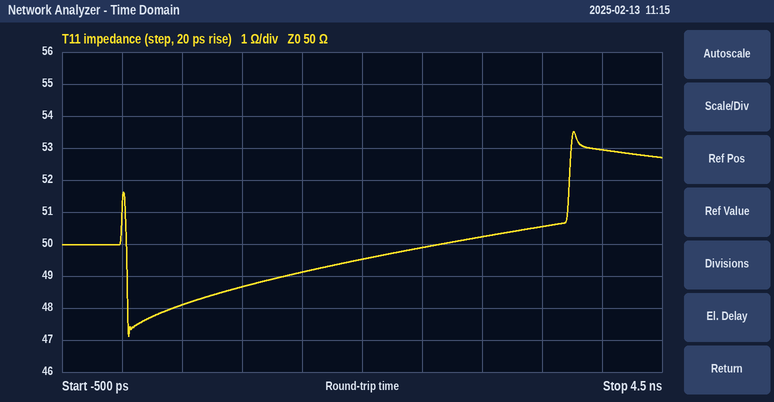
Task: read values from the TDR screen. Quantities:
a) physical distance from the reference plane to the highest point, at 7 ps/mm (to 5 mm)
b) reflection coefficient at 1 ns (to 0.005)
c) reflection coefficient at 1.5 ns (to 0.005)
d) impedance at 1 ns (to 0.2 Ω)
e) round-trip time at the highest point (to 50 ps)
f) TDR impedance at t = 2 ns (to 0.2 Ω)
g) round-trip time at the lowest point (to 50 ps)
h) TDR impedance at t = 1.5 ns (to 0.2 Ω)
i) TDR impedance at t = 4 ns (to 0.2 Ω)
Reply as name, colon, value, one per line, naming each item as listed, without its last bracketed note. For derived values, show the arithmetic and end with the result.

physical distance from the reference plane to the highest point, at 7 ps/mm: 3.75 ns / 2 / 7 ps/mm ≈ 268 mm, so 270 mm to the nearest 5 mm
reflection coefficient at 1 ns: (48.6 − 50)/(48.6 + 50) ≈ -0.0142, so -0.015 to the nearest 0.005
reflection coefficient at 1.5 ns: (49.2 − 50)/(49.2 + 50) ≈ -0.00806, so -0.010 to the nearest 0.005
impedance at 1 ns: 48.6 Ω
round-trip time at the highest point: 3.75 ns
TDR impedance at t = 2 ns: 49.6 Ω
round-trip time at the lowest point: 50 ps
TDR impedance at t = 1.5 ns: 49.2 Ω
TDR impedance at t = 4 ns: 53.0 Ω
